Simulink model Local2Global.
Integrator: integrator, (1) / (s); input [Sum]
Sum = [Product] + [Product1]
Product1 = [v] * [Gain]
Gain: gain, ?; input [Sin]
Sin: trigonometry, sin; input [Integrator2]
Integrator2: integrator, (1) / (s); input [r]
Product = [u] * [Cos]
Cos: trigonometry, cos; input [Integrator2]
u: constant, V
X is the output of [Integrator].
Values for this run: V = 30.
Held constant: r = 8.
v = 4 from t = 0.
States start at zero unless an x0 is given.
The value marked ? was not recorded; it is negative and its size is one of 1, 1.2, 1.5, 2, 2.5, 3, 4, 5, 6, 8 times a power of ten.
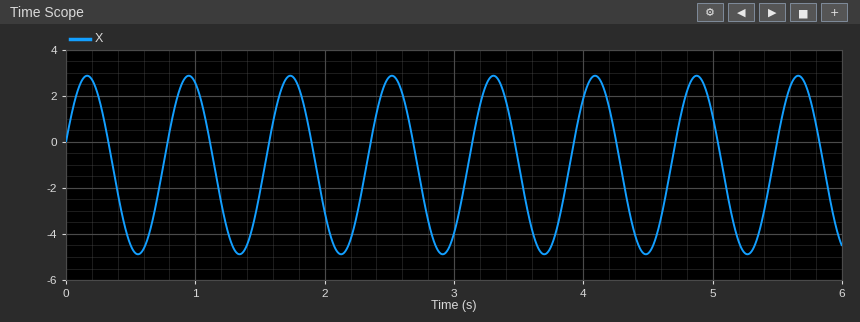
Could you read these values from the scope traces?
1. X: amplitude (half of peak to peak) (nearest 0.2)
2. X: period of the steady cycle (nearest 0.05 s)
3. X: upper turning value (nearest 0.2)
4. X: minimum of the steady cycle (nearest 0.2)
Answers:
3.8
0.80 s
2.8
-4.8
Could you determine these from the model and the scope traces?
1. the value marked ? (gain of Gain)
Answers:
-2
